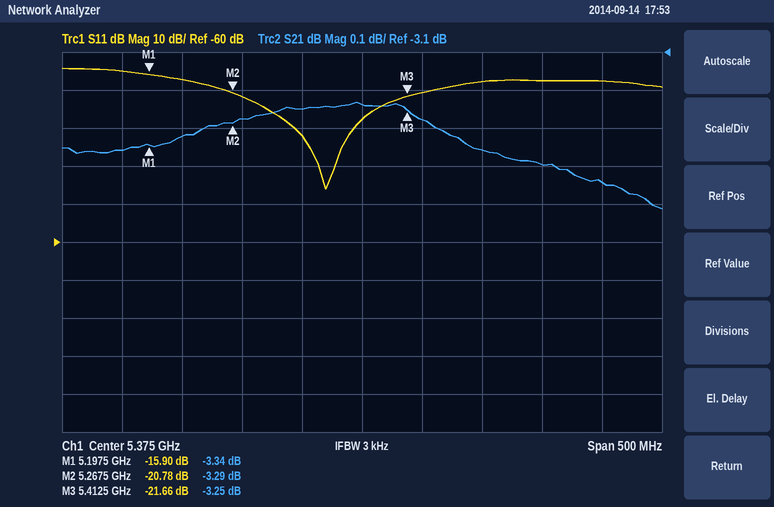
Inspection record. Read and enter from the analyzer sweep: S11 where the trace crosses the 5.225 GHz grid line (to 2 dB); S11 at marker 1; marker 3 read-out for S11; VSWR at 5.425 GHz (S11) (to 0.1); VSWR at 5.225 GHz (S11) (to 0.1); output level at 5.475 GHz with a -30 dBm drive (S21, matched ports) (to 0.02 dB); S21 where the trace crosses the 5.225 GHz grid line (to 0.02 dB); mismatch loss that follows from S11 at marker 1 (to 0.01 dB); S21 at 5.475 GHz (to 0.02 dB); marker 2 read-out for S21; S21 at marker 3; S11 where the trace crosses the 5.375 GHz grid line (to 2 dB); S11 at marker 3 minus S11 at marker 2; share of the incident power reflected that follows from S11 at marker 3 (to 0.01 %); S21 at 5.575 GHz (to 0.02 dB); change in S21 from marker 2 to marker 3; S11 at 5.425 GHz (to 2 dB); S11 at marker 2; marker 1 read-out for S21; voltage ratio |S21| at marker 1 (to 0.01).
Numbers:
-18 dB
-15.90 dB
-21.66 dB
1.2
1.3
-33.36 dBm
-3.32 dB
0.11 dB
-3.36 dB
-3.29 dB
-3.25 dB
-28 dB
-0.88 dB
0.68 %
-3.44 dB
0.04 dB
-20 dB
-20.78 dB
-3.34 dB
0.68
